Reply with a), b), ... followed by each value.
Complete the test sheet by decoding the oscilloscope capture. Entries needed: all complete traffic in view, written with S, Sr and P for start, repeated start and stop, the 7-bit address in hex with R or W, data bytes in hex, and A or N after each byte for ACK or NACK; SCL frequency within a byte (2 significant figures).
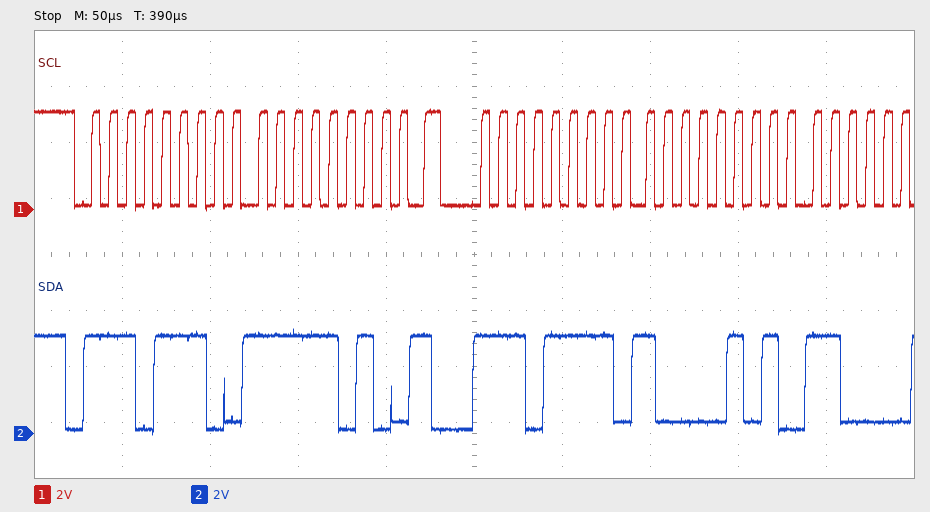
a) S 77W A FA A Sr 77R A 85 A
b) 100 kHz
